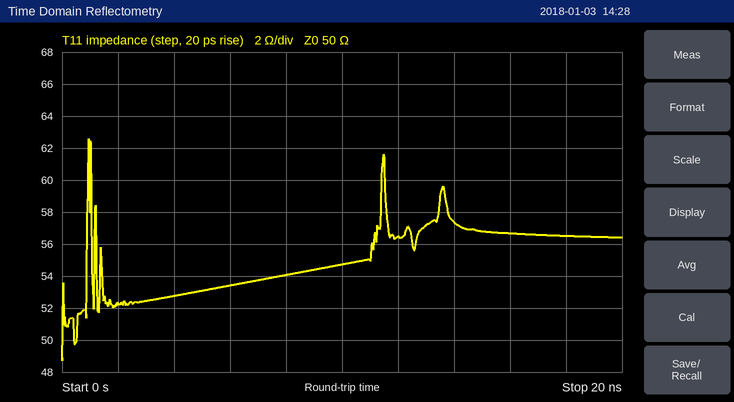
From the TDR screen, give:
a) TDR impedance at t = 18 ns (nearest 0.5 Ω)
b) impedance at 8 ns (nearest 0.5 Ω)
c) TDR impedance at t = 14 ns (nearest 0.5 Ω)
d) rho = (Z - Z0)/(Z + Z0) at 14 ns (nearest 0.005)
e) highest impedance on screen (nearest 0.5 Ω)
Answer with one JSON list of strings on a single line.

["56.5 Ω", "54.0 Ω", "57.5 Ω", "+0.070", "62.5 Ω"]
